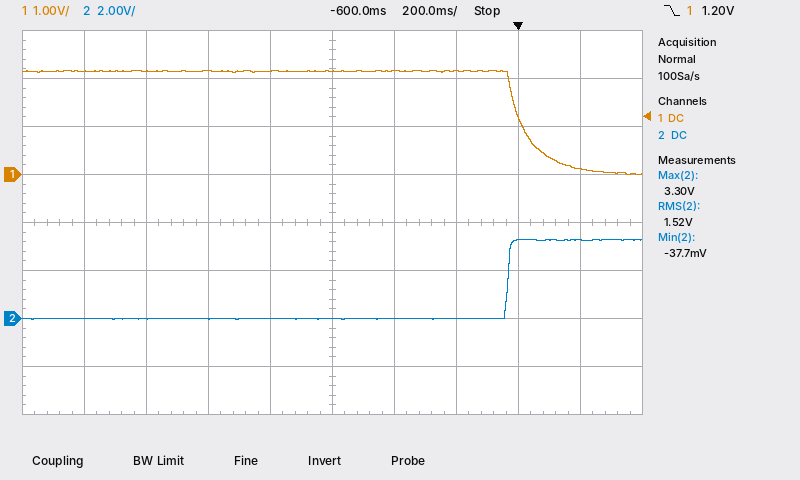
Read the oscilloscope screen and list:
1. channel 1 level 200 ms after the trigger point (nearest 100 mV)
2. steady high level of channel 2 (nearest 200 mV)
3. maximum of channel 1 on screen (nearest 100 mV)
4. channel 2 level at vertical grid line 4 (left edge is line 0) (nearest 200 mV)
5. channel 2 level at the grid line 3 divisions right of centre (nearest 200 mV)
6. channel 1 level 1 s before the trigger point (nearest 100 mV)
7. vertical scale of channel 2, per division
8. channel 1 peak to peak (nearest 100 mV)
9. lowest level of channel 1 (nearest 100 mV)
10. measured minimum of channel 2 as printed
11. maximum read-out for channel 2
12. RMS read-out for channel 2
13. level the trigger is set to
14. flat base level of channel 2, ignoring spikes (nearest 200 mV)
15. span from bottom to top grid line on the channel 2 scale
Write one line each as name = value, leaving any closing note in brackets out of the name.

channel 1 level 200 ms after the trigger point = 100 mV
steady high level of channel 2 = 3.2 V
maximum of channel 1 on screen = 2.2 V
channel 2 level at vertical grid line 4 (left edge is line 0) = 0.0 V
channel 2 level at the grid line 3 divisions right of centre = 3.2 V
channel 1 level 1 s before the trigger point = 2.2 V
vertical scale of channel 2, per division = 2 V
channel 1 peak to peak = 2.2 V
lowest level of channel 1 = 0.0 V
measured minimum of channel 2 as printed = -37.7 mV
maximum read-out for channel 2 = 3.30 V
RMS read-out for channel 2 = 1.52 V
level the trigger is set to = 1.20 V
flat base level of channel 2, ignoring spikes = 0.0 V
span from bottom to top grid line on the channel 2 scale = 16 V
